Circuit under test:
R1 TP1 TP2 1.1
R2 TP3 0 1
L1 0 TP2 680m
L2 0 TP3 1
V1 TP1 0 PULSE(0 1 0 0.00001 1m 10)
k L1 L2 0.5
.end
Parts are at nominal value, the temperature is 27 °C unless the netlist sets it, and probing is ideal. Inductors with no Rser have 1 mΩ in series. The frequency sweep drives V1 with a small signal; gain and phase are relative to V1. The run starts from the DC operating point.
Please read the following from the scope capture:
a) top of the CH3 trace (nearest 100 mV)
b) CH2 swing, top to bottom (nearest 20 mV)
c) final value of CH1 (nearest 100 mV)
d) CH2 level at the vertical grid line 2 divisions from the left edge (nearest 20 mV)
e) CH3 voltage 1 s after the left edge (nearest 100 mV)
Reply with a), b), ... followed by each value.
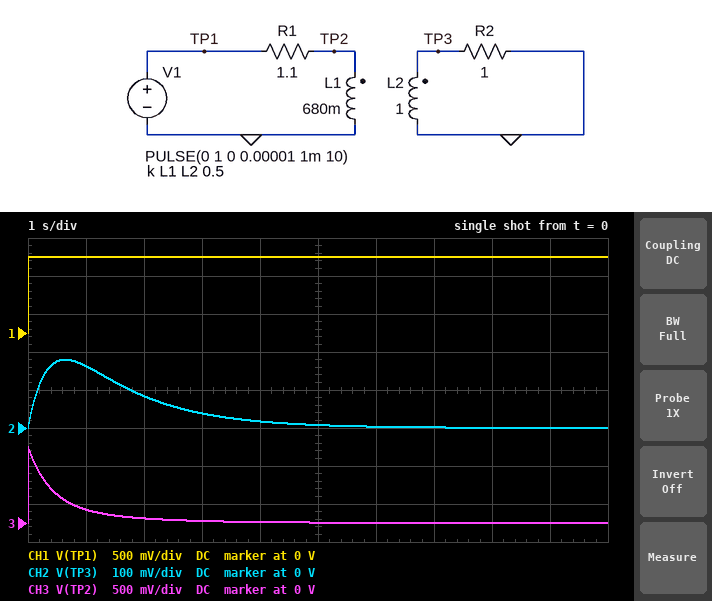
a) 1.0 V
b) 180 mV
c) 1.0 V
d) 80 mV
e) 200 mV
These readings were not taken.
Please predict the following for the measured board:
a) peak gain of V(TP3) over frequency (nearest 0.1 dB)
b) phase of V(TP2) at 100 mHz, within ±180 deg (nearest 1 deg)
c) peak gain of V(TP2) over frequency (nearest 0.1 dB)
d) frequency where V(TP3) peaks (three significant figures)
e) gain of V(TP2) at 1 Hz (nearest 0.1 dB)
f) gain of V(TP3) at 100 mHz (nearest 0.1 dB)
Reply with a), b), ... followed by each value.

a) -12.7 dB
b) 64 deg
c) 0 dB
d) 234 mHz
e) -0.6 dB
f) -14.9 dB
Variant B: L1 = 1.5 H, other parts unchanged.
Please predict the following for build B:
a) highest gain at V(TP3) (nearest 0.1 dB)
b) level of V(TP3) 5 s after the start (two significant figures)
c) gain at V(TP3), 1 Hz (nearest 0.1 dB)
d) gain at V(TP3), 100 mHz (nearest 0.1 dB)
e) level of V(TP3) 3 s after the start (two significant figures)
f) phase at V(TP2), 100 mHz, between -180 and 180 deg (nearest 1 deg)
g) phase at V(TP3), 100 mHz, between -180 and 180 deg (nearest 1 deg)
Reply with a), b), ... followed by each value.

a) -12.6 dB
b) 28 mV
c) -21.6 dB
d) -13.2 dB
e) 83 mV
f) 47 deg
g) 22 deg
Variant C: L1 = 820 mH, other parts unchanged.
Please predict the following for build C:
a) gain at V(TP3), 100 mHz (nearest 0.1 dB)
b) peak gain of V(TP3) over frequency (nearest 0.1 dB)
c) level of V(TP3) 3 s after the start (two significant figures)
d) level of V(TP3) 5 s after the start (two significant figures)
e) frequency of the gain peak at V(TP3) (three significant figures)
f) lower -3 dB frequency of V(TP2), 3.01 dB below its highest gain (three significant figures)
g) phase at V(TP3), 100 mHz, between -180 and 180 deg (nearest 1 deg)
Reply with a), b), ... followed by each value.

a) -14.3 dB
b) -12.6 dB
c) 47 mV
d) 10 mV
e) 213 mHz
f) 299 mHz
g) 35 deg
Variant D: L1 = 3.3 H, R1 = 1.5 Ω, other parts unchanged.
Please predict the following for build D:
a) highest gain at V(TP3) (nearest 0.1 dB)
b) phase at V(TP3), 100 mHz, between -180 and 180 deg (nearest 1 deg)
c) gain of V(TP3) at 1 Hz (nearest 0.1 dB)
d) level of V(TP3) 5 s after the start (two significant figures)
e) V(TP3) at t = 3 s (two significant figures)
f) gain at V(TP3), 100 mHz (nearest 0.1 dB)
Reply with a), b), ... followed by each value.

a) -14.5 dB
b) 10 deg
c) -24.9 dB
d) 45 mV
e) 95 mV
f) -14.6 dB
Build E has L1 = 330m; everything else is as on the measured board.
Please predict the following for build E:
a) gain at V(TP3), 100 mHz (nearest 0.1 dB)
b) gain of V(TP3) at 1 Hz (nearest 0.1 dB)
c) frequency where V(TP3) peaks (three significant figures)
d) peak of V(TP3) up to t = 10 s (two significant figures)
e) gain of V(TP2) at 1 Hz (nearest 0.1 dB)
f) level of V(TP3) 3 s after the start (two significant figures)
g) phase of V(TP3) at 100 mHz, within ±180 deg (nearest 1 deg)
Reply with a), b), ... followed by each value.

a) -17.5 dB
b) -16.8 dB
c) 336 mHz
d) 160 mV
e) -1.9 dB
f) 19 mV
g) 48 deg
